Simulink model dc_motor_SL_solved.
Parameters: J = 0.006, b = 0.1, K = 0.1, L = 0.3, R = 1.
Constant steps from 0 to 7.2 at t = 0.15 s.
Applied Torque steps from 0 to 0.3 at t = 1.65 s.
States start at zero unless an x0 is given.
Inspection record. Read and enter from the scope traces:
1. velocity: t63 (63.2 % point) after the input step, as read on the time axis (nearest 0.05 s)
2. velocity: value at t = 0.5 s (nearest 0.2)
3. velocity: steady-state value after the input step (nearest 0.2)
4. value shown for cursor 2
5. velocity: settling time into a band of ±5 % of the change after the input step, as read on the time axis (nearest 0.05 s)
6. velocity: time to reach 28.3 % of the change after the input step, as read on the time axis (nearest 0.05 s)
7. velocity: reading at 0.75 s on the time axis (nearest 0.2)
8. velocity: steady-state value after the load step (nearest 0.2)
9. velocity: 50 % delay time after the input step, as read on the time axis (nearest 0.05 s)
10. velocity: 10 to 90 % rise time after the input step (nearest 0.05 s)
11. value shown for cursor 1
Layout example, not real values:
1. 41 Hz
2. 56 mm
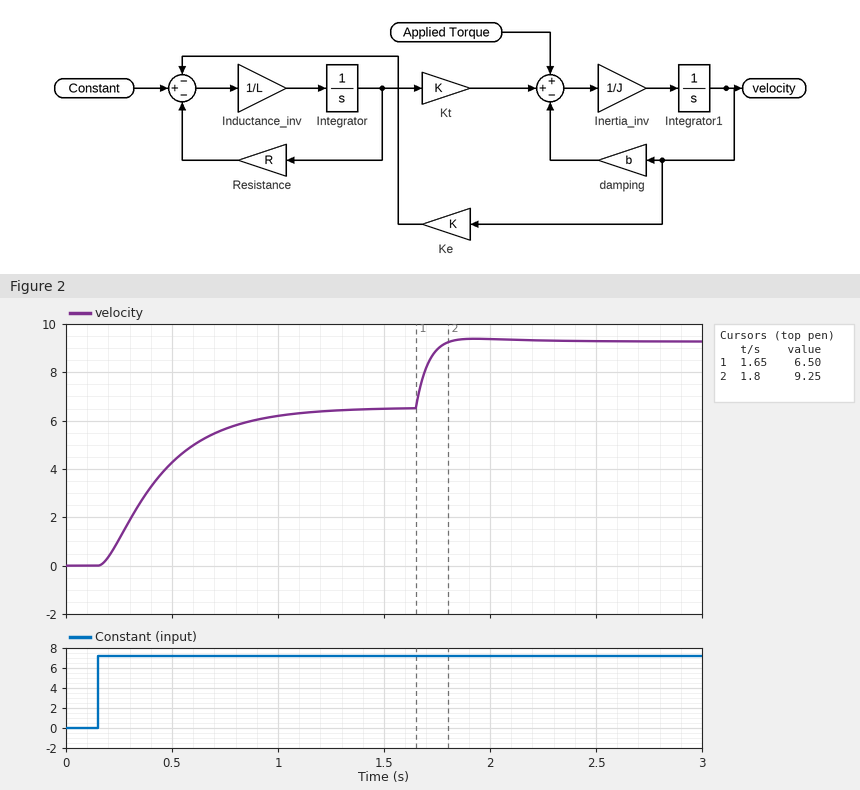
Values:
1. 0.50 s
2. 4.2
3. 6.6
4. 9.25
5. 1.00 s
6. 0.30 s
7. 5.6
8. 9.2
9. 0.40 s
10. 0.60 s
11. 6.50
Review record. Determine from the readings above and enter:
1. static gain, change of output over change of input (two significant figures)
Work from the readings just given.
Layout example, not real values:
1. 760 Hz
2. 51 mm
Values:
1. 0.92
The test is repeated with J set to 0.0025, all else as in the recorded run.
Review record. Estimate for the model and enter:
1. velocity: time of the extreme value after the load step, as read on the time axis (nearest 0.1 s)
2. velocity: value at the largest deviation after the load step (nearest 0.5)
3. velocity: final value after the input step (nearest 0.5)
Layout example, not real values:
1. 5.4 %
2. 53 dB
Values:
1. 1.8 s
2. 9.5
3. 6.5
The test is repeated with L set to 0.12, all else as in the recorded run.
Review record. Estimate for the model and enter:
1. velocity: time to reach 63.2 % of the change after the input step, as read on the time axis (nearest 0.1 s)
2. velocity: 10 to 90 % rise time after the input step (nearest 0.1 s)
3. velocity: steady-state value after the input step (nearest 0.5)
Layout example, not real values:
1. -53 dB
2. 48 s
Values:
1. 0.3 s
2. 0.3 s
3. 6.5
